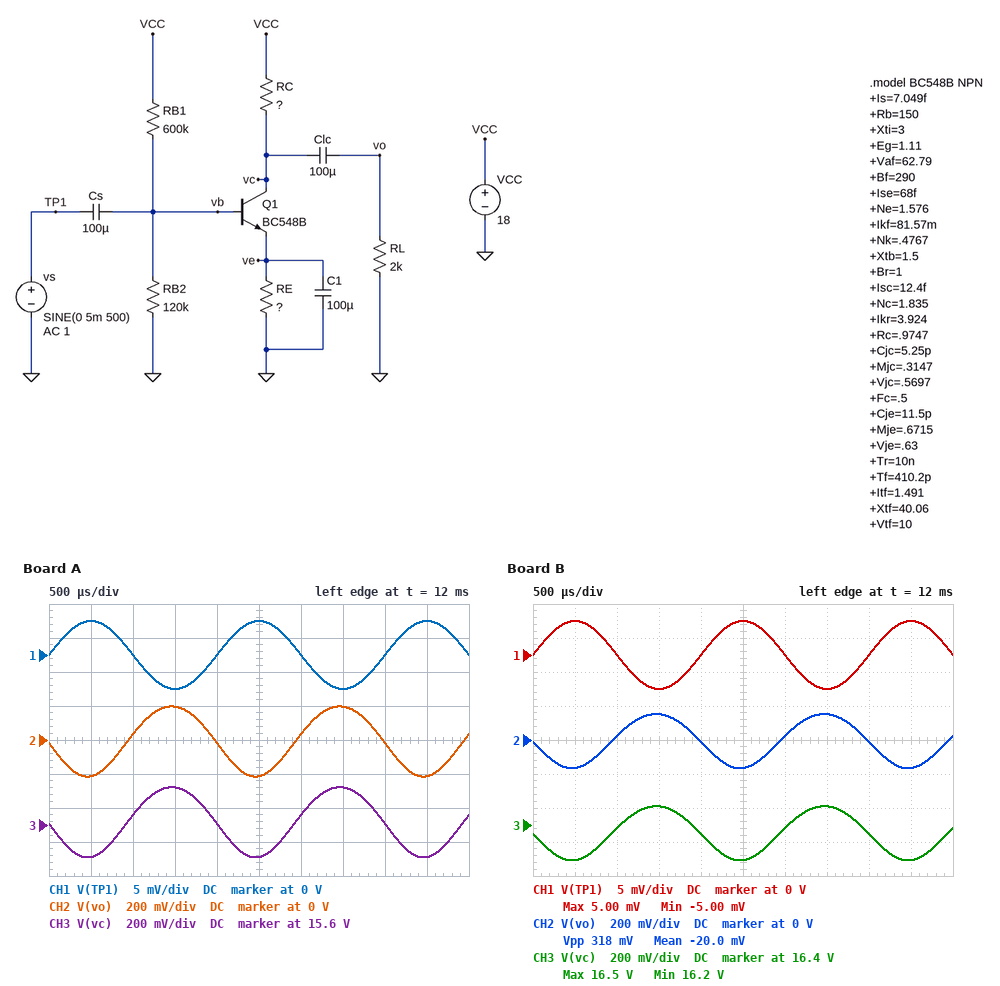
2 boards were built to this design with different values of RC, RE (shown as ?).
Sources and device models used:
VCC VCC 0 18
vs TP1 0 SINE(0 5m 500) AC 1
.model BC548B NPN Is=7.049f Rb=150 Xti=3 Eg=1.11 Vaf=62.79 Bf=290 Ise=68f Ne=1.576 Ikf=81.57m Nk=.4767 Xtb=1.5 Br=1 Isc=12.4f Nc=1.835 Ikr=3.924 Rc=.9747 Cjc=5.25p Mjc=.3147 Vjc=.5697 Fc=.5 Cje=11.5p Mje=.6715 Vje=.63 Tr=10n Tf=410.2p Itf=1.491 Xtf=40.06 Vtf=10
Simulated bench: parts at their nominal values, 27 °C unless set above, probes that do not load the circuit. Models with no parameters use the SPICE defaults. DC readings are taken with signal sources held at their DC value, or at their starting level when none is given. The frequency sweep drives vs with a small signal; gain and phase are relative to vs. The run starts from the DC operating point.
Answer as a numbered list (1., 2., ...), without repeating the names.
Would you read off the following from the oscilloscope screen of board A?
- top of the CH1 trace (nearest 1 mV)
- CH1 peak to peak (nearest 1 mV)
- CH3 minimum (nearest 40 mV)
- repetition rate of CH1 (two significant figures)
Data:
1. 5 mV
2. 10 mV
3. 15.40 V
4. 500 Hz
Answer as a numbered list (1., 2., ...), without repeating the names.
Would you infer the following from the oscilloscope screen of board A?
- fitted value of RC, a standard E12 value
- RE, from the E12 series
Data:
1. 2.2 kΩ
2. 1.8 kΩ
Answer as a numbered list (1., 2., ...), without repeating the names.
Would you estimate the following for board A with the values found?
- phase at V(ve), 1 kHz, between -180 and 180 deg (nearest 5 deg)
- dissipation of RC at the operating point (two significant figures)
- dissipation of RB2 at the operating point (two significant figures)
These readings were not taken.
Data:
1. -85 deg
2. 2.6 mW
3. 57 µW
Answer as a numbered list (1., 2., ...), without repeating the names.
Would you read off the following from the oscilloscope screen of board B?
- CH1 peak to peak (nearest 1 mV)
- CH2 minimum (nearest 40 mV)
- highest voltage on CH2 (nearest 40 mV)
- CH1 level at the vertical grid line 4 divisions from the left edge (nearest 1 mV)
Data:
1. 10 mV
2. -160 mV
3. 160 mV
4. 0 V
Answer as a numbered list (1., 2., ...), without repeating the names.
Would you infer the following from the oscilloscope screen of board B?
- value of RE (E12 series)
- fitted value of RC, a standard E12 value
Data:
1. 2.2 kΩ
2. 1.8 kΩ
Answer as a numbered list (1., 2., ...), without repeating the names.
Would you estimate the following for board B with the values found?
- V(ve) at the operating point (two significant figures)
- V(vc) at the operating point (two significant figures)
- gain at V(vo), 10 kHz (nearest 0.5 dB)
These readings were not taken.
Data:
1. 2.0 V
2. 16 V
3. 30.0 dB
